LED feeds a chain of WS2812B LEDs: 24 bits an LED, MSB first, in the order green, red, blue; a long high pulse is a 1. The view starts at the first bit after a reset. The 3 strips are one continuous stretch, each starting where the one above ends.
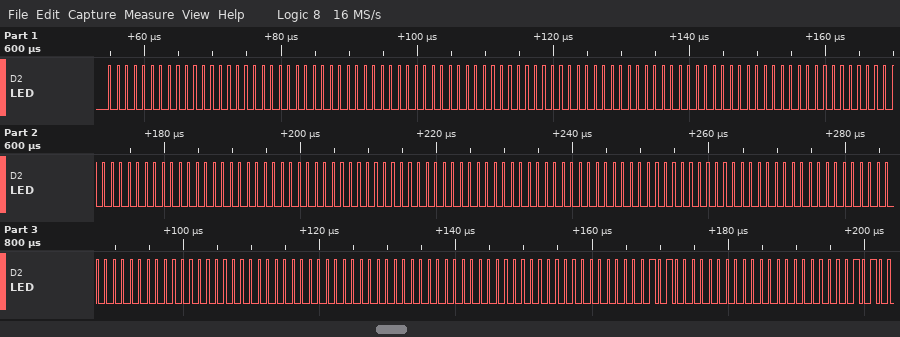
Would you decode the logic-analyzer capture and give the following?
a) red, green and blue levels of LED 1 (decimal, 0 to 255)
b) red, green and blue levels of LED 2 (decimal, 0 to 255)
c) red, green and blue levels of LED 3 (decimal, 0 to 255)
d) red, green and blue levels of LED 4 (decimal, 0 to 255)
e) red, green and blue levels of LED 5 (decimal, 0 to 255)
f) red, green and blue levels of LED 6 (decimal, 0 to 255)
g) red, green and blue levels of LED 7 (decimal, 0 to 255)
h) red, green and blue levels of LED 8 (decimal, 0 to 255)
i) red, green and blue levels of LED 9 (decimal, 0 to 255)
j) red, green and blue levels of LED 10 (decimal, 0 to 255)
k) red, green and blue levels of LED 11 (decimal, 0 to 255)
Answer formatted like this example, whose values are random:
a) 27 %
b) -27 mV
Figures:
a) 0, 0, 0
b) 0, 0, 0
c) 0, 0, 0
d) 0, 0, 0
e) 0, 0, 0
f) 0, 0, 0
g) 0, 0, 0
h) 0, 0, 0
i) 0, 0, 0
j) 0, 0, 0
k) 20, 0, 0
